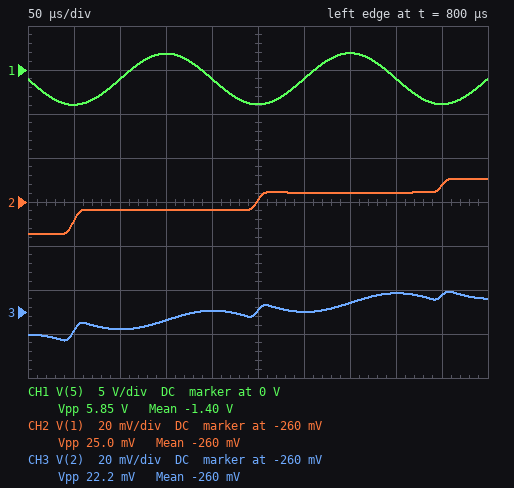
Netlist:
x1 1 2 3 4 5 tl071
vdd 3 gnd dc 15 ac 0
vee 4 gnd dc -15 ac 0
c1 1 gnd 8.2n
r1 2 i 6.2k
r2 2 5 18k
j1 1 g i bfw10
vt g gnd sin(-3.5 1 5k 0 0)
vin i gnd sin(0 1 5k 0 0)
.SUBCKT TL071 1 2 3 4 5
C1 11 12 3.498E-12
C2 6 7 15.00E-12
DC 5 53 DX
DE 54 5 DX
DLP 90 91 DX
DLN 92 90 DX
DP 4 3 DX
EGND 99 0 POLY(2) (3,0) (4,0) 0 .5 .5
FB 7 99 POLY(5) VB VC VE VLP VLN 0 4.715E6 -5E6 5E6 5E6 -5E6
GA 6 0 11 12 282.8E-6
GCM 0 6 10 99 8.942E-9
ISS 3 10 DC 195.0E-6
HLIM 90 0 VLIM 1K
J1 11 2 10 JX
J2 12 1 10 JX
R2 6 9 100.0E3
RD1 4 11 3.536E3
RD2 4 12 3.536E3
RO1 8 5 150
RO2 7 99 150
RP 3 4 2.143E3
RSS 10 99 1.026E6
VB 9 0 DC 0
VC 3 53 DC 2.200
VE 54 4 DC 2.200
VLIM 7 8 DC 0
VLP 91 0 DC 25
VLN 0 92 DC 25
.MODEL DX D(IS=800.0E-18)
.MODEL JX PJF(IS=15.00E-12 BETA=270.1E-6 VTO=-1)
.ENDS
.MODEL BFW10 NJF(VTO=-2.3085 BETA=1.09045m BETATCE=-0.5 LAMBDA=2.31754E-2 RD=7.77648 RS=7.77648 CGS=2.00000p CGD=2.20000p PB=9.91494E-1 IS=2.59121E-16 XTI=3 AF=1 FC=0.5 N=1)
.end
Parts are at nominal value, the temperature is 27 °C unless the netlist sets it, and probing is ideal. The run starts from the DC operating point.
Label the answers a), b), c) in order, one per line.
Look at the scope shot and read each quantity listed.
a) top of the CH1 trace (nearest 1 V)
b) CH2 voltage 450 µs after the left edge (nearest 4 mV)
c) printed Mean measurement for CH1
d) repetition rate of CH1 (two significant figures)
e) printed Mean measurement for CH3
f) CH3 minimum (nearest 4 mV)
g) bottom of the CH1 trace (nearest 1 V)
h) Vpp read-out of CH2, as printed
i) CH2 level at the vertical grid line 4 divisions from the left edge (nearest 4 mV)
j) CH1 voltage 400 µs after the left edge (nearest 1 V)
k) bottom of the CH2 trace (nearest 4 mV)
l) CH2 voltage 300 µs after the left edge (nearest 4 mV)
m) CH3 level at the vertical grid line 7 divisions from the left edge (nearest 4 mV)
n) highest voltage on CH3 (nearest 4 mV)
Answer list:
a) 2 V
b) -252 mV
c) -1.40 V
d) 5.0 kHz
e) -260 mV
f) -272 mV
g) -4 V
h) 25.0 mV
i) -264 mV
j) -1 V
k) -276 mV
l) -256 mV
m) -256 mV
n) -252 mV
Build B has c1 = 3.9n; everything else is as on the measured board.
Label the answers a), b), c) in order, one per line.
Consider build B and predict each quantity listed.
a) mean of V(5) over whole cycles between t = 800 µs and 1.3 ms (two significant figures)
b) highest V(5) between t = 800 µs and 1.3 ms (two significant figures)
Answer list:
a) -920 mV
b) 2.0 V
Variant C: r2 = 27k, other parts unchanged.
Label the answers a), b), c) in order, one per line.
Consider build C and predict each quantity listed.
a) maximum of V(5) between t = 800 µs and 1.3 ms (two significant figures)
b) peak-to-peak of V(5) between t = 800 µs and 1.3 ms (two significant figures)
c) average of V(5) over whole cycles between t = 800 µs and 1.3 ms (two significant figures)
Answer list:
a) 3.0 V
b) 8.8 V
c) -1.4 V
